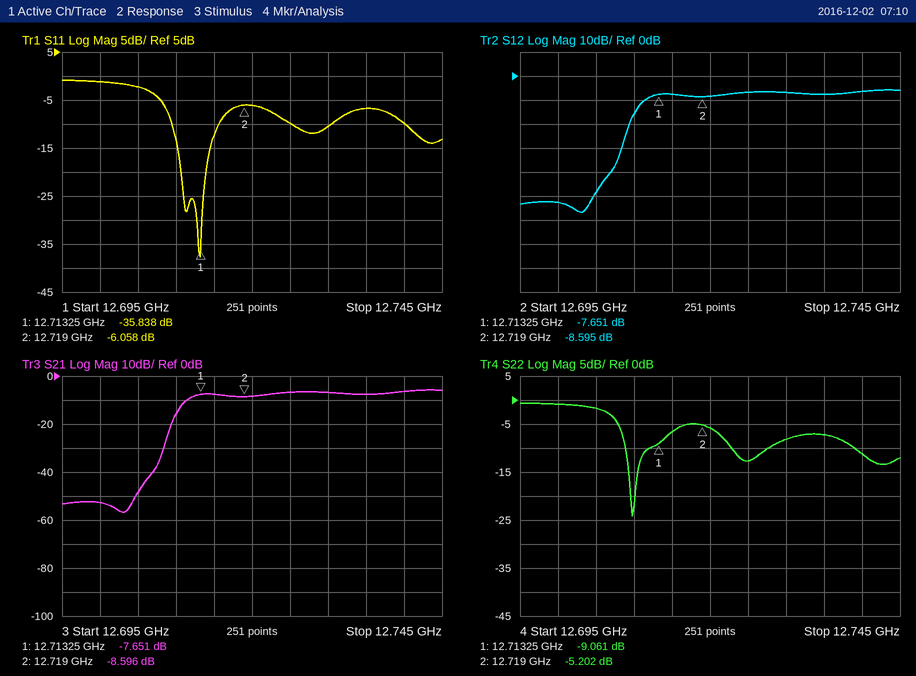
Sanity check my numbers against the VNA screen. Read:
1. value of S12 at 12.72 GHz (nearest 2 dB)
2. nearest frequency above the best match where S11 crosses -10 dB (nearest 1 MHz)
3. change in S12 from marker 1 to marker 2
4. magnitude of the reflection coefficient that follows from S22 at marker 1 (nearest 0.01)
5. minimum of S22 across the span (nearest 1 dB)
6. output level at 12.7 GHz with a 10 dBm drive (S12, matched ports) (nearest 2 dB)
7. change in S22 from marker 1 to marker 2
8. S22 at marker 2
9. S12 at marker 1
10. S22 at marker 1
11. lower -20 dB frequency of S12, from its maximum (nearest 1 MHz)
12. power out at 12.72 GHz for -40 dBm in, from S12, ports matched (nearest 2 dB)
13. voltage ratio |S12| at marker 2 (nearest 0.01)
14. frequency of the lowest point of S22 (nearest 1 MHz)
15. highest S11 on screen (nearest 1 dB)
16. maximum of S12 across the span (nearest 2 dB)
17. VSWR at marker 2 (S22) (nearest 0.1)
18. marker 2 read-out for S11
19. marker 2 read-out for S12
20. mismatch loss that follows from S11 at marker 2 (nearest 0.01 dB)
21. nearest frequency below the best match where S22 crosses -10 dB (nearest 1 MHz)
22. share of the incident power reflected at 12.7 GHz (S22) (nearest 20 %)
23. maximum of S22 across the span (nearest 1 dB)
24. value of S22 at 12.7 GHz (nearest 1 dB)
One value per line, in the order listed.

-8 dB
12.716 GHz
-0.944 dB
0.35
-24 dB
-42 dBm
3.859 dB
-5.202 dB
-7.651 dB
-9.061 dB
12.709 GHz
-48 dBm
0.37
12.710 GHz
-1 dB
-6 dB
3.4
-6.058 dB
-8.595 dB
1.24 dB
12.709 GHz
80 %
-1 dB
-1 dB
